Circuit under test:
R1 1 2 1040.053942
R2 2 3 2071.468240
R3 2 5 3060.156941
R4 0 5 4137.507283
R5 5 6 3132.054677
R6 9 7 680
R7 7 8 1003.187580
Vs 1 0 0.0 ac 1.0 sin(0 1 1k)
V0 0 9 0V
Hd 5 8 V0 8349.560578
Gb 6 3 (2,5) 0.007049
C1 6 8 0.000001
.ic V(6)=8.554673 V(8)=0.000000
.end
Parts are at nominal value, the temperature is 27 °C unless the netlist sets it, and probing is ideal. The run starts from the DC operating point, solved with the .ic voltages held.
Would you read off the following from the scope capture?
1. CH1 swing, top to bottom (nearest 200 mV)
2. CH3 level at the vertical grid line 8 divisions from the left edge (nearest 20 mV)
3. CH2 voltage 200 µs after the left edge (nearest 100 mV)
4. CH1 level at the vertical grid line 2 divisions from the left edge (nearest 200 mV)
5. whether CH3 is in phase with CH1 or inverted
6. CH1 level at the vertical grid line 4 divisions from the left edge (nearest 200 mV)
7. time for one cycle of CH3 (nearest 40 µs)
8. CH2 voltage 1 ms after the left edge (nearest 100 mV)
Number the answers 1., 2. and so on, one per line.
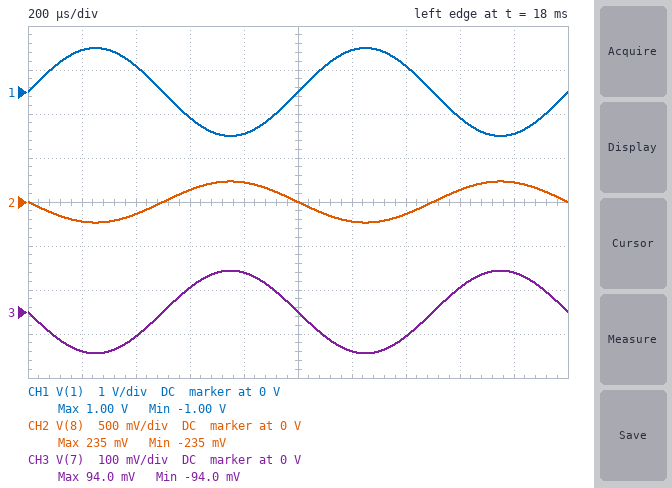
1. 2.0 V
2. 60 mV
3. -200 mV
4. 600 mV
5. inverted
6. -1.0 V
7. 1.00 ms
8. 0 V
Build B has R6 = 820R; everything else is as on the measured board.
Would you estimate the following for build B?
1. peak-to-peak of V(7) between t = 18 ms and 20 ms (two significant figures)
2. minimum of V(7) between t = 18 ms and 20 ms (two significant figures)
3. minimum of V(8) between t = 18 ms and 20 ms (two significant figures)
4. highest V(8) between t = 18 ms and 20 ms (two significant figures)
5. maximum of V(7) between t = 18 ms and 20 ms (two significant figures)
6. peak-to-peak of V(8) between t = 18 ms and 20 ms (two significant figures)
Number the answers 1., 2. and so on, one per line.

1. 230 mV
2. -120 mV
3. -260 mV
4. 260 mV
5. 120 mV
6. 520 mV
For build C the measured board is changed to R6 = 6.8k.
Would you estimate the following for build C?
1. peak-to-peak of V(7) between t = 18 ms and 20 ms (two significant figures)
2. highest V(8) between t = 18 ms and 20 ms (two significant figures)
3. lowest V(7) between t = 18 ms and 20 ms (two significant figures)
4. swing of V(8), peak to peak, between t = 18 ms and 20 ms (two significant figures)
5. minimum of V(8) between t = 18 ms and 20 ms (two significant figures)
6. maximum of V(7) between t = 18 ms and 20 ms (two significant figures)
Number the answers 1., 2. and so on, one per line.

1. 60 V
2. 34 V
3. -30 V
4. 69 V
5. -34 V
6. 30 V
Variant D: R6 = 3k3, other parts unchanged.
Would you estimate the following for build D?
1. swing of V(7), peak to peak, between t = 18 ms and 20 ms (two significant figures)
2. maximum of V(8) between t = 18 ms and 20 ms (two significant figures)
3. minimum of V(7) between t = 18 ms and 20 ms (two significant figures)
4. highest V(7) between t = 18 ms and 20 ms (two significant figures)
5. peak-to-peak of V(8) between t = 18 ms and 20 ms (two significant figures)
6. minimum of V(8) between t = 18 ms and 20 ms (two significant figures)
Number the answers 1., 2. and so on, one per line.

1. 1.6 V
2. 1.1 V
3. -820 mV
4. 820 mV
5. 2.1 V
6. -1.1 V
